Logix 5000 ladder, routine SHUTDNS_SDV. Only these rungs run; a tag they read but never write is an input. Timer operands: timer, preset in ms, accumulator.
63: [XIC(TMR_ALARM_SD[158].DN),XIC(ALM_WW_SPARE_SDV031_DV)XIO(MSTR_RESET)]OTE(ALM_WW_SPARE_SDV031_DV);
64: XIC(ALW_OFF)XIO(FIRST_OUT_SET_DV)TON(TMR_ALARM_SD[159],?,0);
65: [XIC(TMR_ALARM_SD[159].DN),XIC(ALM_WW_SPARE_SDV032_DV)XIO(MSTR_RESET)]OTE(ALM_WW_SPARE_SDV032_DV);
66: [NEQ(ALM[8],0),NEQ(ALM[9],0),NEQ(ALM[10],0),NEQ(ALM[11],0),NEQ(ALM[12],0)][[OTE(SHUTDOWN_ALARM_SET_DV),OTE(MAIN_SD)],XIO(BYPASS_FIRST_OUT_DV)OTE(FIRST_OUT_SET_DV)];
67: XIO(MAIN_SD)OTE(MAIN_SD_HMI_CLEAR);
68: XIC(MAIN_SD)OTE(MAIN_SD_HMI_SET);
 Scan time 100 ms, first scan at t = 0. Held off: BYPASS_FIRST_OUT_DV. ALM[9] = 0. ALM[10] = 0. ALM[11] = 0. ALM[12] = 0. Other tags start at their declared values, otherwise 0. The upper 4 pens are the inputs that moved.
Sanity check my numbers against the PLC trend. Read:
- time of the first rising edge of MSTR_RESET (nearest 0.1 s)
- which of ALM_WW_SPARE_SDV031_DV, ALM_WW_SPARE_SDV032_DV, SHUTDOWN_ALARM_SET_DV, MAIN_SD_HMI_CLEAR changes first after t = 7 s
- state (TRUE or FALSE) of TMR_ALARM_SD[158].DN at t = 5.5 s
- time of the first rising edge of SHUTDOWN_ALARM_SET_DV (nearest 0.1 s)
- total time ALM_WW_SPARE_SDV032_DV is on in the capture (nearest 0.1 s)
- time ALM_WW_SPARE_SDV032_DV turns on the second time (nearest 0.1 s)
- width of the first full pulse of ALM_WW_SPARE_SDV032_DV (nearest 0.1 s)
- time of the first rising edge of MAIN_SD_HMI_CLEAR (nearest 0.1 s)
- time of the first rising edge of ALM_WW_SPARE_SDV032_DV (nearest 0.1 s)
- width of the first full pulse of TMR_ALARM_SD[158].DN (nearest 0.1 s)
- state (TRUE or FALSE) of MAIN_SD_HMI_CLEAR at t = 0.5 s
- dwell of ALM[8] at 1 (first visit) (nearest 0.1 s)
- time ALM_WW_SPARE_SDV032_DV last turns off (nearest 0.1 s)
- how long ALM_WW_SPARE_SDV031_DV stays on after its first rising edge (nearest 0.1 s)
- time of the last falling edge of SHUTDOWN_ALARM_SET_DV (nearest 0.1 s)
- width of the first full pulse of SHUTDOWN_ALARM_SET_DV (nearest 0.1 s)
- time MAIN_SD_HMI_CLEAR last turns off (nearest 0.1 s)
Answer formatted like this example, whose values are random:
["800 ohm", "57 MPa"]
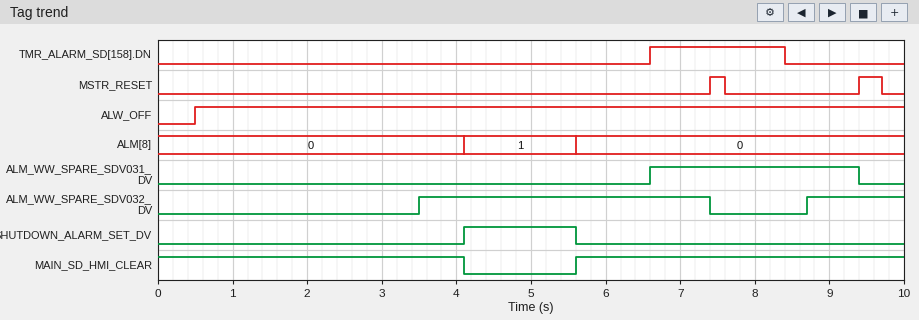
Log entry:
["7.4 s", "ALM_WW_SPARE_SDV032_DV", "FALSE", "4.1 s", "5.2 s", "8.7 s", "3.9 s", "5.6 s", "3.5 s", "1.8 s", "TRUE", "1.5 s", "7.4 s", "2.8 s", "5.6 s", "1.5 s", "4.1 s"]
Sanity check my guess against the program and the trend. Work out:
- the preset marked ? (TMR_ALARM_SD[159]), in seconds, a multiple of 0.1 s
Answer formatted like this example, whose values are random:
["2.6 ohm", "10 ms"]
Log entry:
["3.0 s"]
